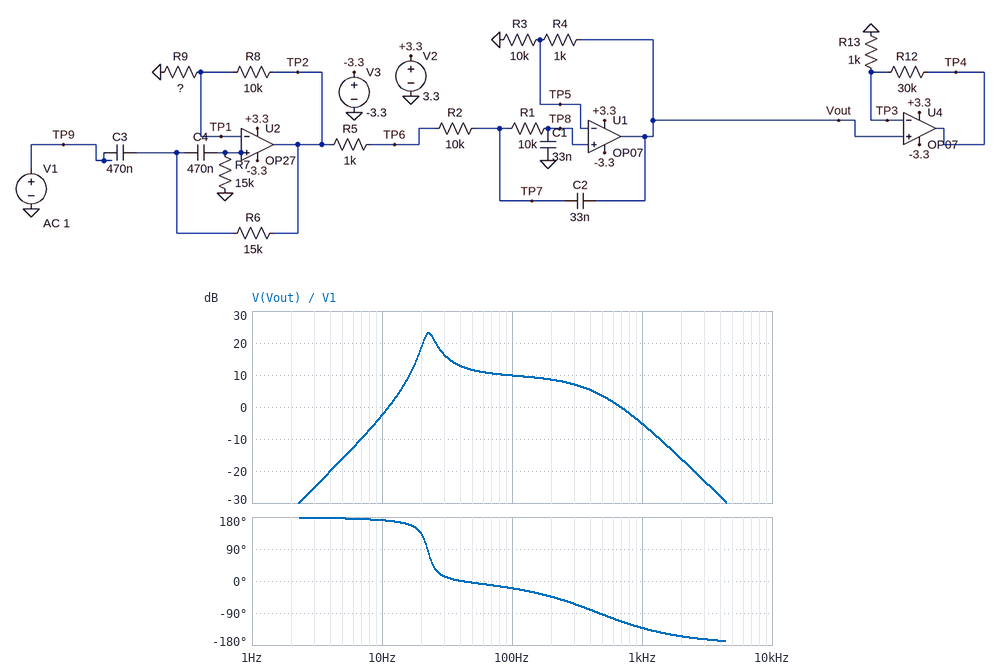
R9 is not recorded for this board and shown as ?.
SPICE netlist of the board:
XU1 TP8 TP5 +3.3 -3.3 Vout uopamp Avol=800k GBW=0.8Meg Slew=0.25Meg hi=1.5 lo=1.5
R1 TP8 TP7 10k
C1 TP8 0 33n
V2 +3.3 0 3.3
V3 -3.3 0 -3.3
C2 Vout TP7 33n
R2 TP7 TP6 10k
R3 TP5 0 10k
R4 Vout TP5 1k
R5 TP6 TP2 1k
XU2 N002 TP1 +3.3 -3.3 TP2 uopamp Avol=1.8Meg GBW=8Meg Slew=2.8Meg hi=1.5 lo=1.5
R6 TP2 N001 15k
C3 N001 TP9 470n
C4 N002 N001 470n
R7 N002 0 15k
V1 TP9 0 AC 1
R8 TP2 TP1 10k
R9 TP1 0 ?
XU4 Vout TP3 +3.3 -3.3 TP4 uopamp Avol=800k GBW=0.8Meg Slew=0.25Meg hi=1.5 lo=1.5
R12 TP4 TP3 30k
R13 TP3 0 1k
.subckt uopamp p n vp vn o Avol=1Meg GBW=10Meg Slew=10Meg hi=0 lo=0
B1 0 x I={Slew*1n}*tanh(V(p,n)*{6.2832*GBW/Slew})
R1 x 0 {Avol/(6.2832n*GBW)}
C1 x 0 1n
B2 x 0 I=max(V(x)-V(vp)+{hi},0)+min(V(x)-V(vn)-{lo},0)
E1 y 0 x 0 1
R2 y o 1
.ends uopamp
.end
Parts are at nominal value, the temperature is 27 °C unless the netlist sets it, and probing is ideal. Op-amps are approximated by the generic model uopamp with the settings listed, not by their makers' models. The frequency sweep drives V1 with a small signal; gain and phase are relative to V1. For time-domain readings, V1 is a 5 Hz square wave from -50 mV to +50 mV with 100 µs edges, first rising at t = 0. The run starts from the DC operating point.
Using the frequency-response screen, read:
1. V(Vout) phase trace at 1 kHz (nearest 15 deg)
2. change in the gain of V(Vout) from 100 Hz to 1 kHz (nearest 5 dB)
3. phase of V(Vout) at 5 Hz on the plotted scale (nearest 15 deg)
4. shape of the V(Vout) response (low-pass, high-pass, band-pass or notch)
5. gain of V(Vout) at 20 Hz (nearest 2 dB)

-135 deg
-15 dB
180 deg
band-pass
18 dB
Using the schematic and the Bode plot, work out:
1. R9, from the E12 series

5.6 kΩ
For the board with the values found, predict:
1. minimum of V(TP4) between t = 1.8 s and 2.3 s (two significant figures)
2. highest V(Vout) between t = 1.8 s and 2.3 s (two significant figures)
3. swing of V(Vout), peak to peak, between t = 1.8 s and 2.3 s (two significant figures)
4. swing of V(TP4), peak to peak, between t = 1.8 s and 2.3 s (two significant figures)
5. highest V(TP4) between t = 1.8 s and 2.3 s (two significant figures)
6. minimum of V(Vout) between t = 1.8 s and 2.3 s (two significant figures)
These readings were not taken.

-1.8 V
290 mV
580 mV
3.6 V
1.8 V
-290 mV
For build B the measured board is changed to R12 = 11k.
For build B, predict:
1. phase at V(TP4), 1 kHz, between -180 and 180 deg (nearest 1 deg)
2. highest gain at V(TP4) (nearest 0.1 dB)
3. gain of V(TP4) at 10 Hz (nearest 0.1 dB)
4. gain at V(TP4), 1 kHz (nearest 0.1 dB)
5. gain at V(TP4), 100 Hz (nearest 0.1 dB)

-133 deg
44.7 dB
19.0 dB
16.4 dB
31.4 dB
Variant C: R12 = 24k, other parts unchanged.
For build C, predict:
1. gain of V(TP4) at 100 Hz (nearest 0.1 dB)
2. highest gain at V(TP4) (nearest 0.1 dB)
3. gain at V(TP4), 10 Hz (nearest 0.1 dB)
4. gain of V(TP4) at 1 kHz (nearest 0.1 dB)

37.8 dB
51.1 dB
25.4 dB
22.8 dB
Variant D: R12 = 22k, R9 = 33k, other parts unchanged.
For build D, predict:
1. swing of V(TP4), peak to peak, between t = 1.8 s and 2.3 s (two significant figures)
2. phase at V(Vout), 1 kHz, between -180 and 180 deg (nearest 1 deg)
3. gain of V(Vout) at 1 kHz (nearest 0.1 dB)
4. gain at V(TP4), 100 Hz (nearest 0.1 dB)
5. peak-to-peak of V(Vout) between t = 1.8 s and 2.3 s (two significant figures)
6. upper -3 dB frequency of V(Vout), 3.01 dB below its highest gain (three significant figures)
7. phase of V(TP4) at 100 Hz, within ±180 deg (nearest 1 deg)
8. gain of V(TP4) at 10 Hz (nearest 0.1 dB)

3.6 V
-130 deg
-11.8 dB
29.8 dB
220 mV
348 Hz
-2 deg
15.4 dB
